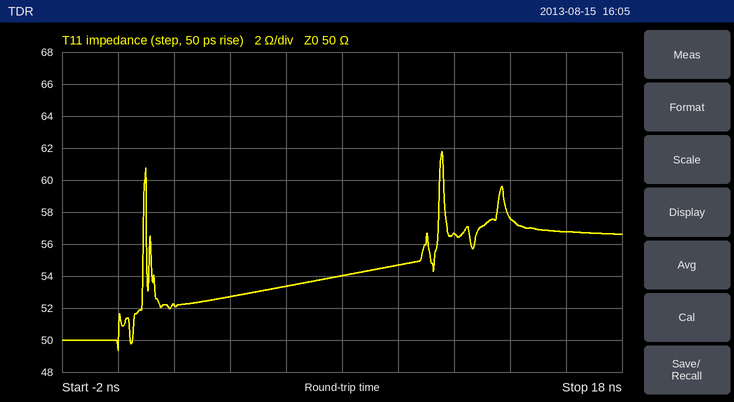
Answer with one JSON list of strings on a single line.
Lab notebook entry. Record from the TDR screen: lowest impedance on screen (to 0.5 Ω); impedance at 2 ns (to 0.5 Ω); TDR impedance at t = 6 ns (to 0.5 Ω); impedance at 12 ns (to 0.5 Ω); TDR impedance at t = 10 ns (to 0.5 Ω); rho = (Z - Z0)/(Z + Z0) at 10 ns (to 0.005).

["49.5 Ω", "52.0 Ω", "53.5 Ω", "56.5 Ω", "54.5 Ω", "+0.045"]
